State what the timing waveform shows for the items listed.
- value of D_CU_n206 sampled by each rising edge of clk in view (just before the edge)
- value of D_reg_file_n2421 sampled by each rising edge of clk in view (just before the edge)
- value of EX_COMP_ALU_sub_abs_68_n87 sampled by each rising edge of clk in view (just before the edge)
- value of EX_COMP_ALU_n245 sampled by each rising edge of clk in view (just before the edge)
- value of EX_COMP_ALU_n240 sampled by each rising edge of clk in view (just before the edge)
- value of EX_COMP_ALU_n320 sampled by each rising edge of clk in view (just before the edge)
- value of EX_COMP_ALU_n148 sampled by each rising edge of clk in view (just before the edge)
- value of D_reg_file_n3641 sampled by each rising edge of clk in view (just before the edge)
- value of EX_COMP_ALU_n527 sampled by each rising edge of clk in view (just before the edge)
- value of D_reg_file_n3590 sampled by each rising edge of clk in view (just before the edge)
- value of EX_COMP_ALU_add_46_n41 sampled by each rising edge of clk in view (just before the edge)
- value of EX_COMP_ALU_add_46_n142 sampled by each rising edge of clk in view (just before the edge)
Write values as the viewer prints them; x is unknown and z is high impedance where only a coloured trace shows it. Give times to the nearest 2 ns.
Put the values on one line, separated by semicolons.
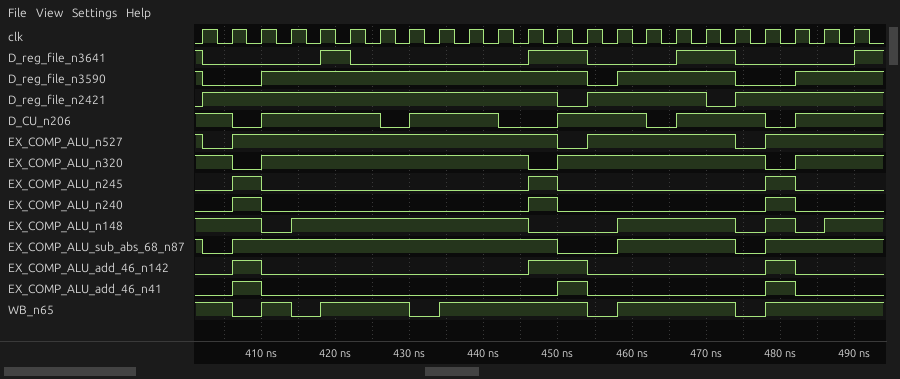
1 1 0 1 1 1 1 0 1 1 1 0 0 1 1 1 0 1 1 1 0 1 1; 0 1 1 1 1 1 1 1 1 1 1 1 1 0 1 1 1 1 0 1 1 1 1; 1 0 1 1 1 1 1 1 1 1 1 1 1 0 0 1 1 1 1 0 1 1 1; 0 0 1 0 0 0 0 0 0 0 0 0 1 0 0 0 0 0 0 0 1 0 0; 0 0 1 0 0 0 0 0 0 0 0 0 1 0 0 0 0 0 0 0 1 0 0; 1 1 0 1 1 1 1 1 1 1 1 1 0 1 1 1 1 1 1 1 0 1 1; 1 1 1 0 1 1 1 1 1 1 1 1 0 0 0 1 1 1 1 0 1 0 1; 1 0 0 0 0 1 0 0 0 0 0 0 1 1 0 0 0 1 1 0 0 0 0; 1 0 1 1 1 1 1 1 1 1 1 1 1 0 1 1 1 1 1 0 1 1 1; 1 0 0 1 1 1 1 1 1 1 1 1 1 1 0 1 1 1 1 0 0 1 1; 0 0 1 0 0 0 0 0 0 0 0 0 0 1 0 0 0 0 0 0 1 0 0; 0 0 1 0 0 0 0 0 0 0 0 0 1 1 0 0 0 0 0 0 1 0 0
